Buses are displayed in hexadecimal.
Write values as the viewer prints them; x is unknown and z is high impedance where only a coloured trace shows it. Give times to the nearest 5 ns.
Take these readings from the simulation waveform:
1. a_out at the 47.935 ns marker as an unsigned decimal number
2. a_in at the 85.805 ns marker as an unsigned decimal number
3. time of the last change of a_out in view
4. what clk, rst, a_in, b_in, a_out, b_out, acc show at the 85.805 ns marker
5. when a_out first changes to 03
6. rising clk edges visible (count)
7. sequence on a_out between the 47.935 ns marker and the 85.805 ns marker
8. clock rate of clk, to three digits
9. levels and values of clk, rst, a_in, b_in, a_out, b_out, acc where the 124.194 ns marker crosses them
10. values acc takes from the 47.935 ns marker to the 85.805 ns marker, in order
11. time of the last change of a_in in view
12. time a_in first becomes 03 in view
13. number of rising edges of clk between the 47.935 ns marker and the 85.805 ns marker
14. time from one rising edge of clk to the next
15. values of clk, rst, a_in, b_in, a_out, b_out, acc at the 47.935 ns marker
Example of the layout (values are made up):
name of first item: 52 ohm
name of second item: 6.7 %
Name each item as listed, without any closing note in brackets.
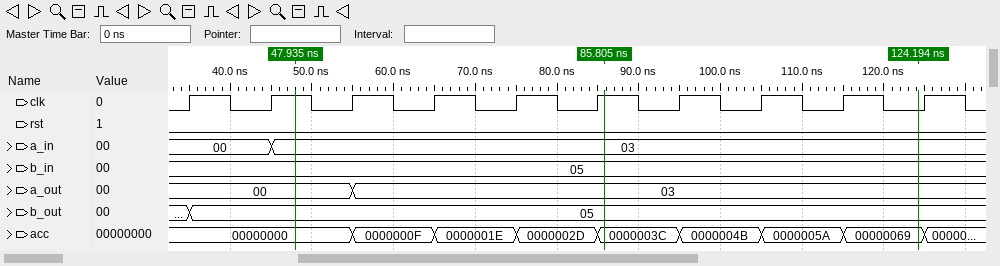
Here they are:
a_out at the 47.935 ns marker as an unsigned decimal number: 0
a_in at the 85.805 ns marker as an unsigned decimal number: 3
time of the last change of a_out in view: 55 ns
what clk, rst, a_in, b_in, a_out, b_out, acc show at the 85.805 ns marker: clk=1, rst=0, a_in=03, b_in=05, a_out=03, b_out=05, acc=0000003C
when a_out first changes to 03: 55 ns
rising clk edges visible: 10
sequence on a_out between the 47.935 ns marker and the 85.805 ns marker: 00, 03
clock rate of clk, to three digits: 100 MHz
levels and values of clk, rst, a_in, b_in, a_out, b_out, acc where the 124.194 ns marker crosses them: clk=0, rst=0, a_in=03, b_in=05, a_out=03, b_out=05, acc=00000069
values acc takes from the 47.935 ns marker to the 85.805 ns marker, in order: 00000000, 0000000F, 0000001E, 0000002D, 0000003C
time of the last change of a_in in view: 45 ns
time a_in first becomes 03 in view: 45 ns
number of rising edges of clk between the 47.935 ns marker and the 85.805 ns marker: 4
time from one rising edge of clk to the next: 10 ns
values of clk, rst, a_in, b_in, a_out, b_out, acc at the 47.935 ns marker: clk=1, rst=0, a_in=03, b_in=05, a_out=00, b_out=05, acc=00000000
